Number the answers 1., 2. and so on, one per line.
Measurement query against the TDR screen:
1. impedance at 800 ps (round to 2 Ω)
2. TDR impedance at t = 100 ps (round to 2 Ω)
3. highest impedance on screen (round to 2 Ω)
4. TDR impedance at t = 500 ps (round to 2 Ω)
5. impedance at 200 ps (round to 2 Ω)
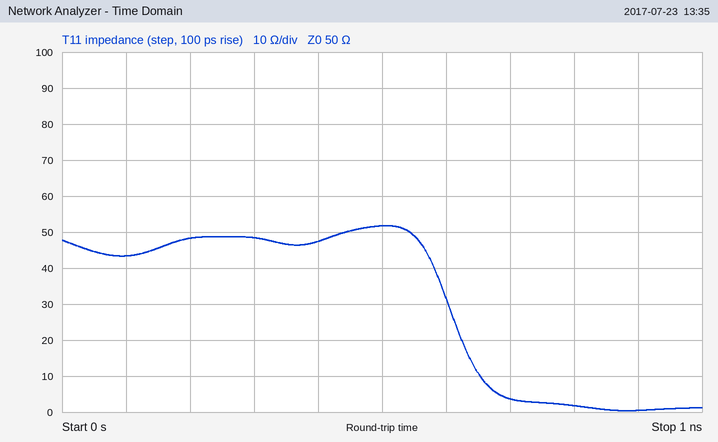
1. 2 Ω
2. 44 Ω
3. 52 Ω
4. 52 Ω
5. 48 Ω
